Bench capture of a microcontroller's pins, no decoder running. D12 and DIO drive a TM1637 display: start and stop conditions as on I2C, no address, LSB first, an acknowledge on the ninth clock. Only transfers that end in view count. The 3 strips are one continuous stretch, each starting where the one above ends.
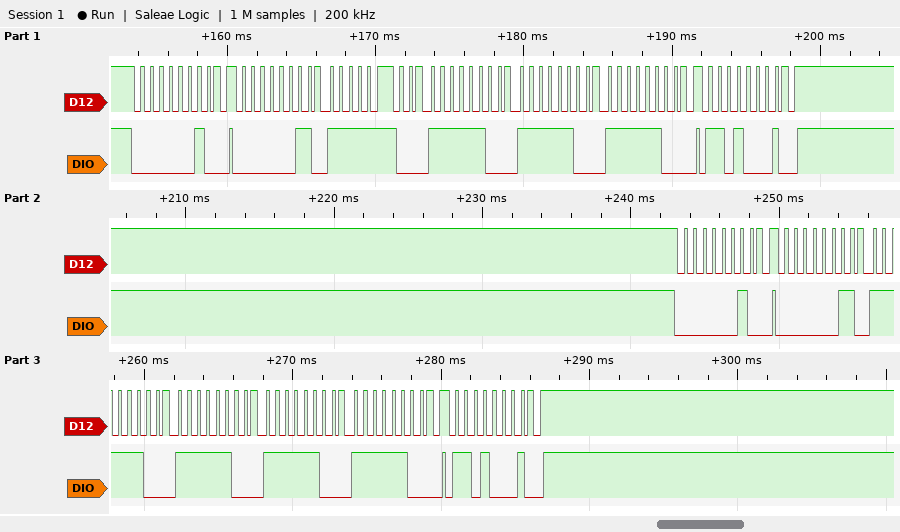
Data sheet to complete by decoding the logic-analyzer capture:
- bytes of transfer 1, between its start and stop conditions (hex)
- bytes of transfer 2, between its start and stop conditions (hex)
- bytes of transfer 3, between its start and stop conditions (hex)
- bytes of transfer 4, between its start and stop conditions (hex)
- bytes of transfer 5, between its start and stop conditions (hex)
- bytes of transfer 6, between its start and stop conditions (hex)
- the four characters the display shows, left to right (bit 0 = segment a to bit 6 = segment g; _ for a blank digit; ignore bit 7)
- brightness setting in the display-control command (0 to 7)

40
C0 3F 3F 3F 3F
8B
40
C0 3F 3F 3F 3F
8B
0000
3
